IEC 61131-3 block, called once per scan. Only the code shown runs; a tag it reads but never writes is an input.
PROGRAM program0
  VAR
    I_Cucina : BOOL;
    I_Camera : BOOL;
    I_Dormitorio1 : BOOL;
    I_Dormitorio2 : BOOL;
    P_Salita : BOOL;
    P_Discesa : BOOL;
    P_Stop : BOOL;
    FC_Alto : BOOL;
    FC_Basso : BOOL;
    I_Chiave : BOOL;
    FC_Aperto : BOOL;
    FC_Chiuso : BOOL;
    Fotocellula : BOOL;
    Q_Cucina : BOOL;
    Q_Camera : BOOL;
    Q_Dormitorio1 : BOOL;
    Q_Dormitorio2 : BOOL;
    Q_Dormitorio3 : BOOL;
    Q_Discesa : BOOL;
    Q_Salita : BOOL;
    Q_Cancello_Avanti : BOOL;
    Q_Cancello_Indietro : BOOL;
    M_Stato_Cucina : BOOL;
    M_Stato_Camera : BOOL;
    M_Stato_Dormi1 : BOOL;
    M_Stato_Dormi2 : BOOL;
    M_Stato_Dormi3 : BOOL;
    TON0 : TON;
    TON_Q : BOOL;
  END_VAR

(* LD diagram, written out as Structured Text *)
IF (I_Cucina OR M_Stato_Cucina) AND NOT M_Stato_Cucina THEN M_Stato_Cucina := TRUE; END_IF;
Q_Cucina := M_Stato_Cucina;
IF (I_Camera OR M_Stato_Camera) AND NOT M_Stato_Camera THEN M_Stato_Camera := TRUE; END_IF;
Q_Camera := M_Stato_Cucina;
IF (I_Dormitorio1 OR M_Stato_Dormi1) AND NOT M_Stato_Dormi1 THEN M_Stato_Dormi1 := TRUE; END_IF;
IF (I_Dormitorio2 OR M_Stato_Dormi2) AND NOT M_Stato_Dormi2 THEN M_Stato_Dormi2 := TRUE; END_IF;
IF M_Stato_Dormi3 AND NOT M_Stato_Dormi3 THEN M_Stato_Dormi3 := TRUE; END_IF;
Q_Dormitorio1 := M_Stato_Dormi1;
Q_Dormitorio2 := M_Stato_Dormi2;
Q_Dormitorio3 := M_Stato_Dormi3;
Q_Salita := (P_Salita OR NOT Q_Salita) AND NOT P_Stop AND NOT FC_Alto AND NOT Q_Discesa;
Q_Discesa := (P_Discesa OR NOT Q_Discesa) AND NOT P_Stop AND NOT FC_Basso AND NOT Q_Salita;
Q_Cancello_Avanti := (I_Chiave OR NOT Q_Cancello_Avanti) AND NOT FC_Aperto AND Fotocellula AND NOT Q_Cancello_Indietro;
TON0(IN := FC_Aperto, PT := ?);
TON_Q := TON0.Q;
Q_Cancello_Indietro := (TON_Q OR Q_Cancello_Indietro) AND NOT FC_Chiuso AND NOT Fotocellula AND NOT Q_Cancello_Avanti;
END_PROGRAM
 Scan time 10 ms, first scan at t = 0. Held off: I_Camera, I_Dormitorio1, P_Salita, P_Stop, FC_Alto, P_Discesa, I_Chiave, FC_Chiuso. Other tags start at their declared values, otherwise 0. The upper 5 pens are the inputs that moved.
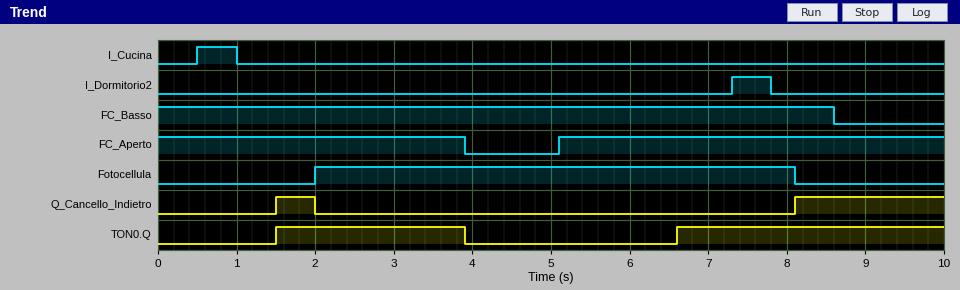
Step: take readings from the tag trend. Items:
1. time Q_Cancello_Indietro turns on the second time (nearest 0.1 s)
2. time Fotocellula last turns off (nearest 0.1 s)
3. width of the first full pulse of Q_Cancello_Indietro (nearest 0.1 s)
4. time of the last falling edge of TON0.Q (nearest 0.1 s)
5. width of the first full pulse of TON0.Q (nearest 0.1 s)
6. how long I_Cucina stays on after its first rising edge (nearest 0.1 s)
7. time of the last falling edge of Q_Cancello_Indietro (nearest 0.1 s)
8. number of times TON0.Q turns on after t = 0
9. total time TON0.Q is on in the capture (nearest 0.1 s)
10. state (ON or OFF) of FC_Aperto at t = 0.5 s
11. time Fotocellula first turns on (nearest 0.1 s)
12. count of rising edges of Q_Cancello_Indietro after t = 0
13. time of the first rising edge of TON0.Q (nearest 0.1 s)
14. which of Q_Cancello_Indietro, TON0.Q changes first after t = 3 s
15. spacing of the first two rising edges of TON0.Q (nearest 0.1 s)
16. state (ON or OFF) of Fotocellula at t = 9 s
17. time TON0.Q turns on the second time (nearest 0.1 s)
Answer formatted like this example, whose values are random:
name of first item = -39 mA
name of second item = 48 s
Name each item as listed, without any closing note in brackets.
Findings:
time Q_Cancello_Indietro turns on the second time = 8.1 s
time Fotocellula last turns off = 8.1 s
width of the first full pulse of Q_Cancello_Indietro = 0.5 s
time of the last falling edge of TON0.Q = 3.9 s
width of the first full pulse of TON0.Q = 2.4 s
how long I_Cucina stays on after its first rising edge = 0.5 s
time of the last falling edge of Q_Cancello_Indietro = 2.0 s
number of times TON0.Q turns on after t = 0 = 2
total time TON0.Q is on in the capture = 5.8 s
state (ON or OFF) of FC_Aperto at t = 0.5 s = ON
time Fotocellula first turns on = 2.0 s
count of rising edges of Q_Cancello_Indietro after t = 0 = 2
time of the first rising edge of TON0.Q = 1.5 s
which of Q_Cancello_Indietro, TON0.Q changes first after t = 3 s = TON0.Q
spacing of the first two rising edges of TON0.Q = 5.1 s
state (ON or OFF) of Fotocellula at t = 9 s = OFF
time TON0.Q turns on the second time = 6.6 s
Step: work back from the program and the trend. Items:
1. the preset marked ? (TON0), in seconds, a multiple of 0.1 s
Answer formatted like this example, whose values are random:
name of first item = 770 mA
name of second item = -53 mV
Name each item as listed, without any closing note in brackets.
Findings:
the preset marked ? (TON0), in seconds, a multiple of 0.1 s = 1.5 s
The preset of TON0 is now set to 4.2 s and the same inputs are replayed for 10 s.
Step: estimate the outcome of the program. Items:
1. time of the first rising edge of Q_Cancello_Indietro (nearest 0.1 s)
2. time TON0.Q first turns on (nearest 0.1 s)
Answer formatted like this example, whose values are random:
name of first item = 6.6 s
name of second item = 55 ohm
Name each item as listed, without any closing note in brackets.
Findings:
time of the first rising edge of Q_Cancello_Indietro = 9.3 s
time TON0.Q first turns on = 9.3 s
